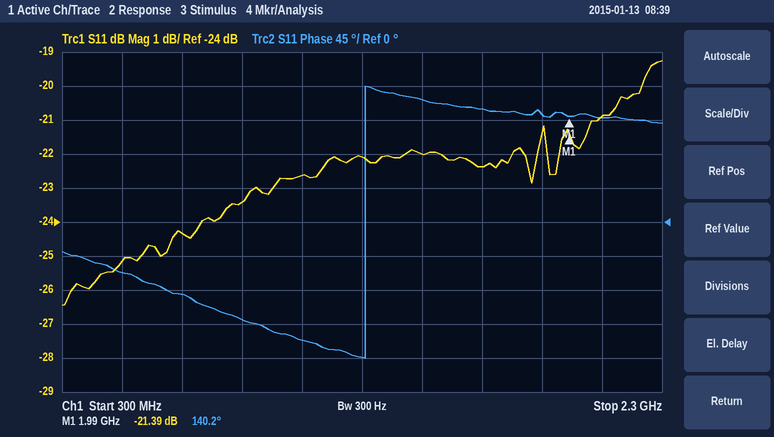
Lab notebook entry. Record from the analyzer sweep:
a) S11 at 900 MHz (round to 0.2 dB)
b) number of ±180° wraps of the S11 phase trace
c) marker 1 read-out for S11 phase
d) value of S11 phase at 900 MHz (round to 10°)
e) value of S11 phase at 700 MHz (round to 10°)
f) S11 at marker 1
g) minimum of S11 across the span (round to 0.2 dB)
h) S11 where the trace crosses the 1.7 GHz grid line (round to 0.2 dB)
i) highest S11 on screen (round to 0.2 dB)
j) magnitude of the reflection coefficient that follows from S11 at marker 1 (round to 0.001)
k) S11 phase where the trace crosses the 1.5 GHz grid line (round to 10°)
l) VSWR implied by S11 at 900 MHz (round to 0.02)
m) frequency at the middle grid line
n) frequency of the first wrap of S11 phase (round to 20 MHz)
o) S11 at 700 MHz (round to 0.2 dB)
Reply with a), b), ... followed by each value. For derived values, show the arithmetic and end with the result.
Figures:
a) -23.4 dB
b) 1
c) 140.2°
d) -130°
e) -100°
f) -21.39 dB
g) -26.4 dB
h) -22.4 dB
i) -19.2 dB
j) 10^(-21.39/20) ≈ 0.085
k) 160°
l) |Γ| = 10^(-23.4/20) = 0.0676; VSWR = (1 + 0.0676)/(1 − 0.0676) ≈ 1.15, so 1.14 to the nearest 0.02
m) 1.3 GHz
n) 1.32 GHz
o) -24.4 dB
